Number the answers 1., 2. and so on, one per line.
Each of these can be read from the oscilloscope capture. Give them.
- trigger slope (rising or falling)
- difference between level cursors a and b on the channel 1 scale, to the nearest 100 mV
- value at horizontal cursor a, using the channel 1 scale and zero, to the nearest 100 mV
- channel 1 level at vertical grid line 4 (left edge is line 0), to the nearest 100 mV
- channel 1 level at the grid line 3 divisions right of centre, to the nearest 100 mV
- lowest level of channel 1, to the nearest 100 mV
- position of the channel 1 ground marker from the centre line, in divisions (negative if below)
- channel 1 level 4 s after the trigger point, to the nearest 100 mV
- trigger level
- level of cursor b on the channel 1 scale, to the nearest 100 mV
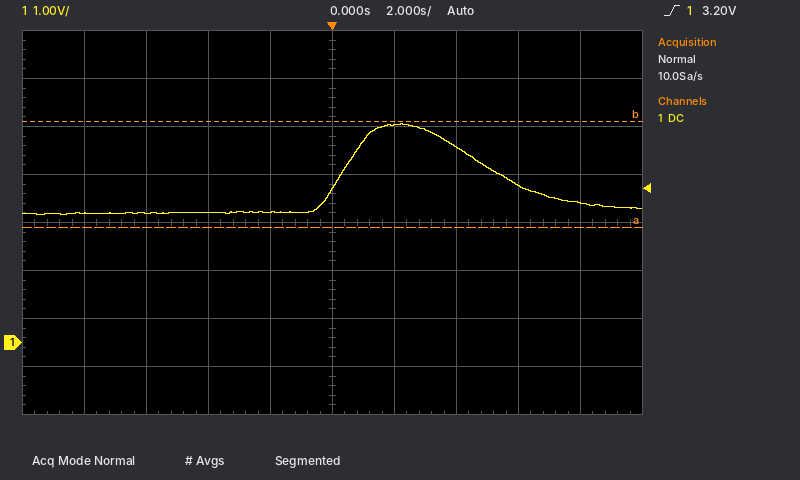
1. rising
2. 2.2 V
3. 2.4 V
4. 2.7 V
5. 3.3 V
6. 2.7 V
7. -2.5 div
8. 4.1 V
9. 3.20 V
10. 4.6 V
